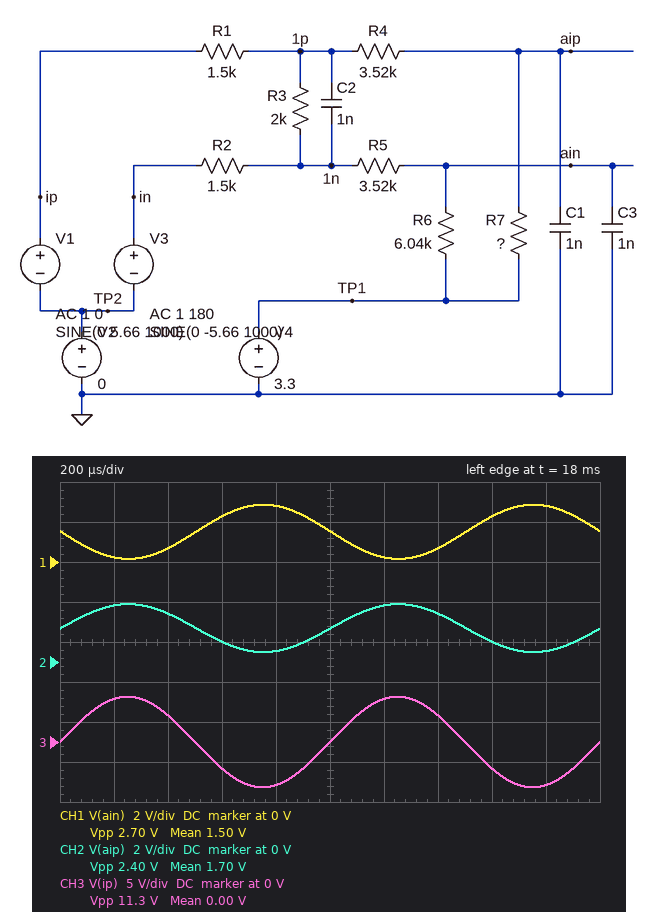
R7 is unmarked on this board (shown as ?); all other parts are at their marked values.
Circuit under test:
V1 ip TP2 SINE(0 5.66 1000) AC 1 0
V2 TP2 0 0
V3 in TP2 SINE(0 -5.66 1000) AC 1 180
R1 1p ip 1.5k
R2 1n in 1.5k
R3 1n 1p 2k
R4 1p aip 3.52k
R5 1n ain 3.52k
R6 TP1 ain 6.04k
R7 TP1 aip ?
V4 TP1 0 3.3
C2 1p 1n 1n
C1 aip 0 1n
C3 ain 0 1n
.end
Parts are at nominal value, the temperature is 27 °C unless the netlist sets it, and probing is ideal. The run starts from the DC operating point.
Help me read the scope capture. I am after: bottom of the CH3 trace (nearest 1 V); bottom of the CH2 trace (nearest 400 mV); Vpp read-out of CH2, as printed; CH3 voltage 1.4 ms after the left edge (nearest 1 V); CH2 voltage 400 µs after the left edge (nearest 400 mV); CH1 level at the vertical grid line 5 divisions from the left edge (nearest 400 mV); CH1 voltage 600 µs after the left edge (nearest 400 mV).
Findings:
-6 V
400 mV
2.40 V
3 V
2.4 V
1.6 V
2.4 V
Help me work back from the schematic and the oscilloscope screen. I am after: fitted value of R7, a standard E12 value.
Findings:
4.7 kΩ
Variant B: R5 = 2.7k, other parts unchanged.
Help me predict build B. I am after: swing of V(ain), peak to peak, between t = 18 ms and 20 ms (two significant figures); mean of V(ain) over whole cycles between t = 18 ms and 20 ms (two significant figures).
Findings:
2.9 V
1.4 V
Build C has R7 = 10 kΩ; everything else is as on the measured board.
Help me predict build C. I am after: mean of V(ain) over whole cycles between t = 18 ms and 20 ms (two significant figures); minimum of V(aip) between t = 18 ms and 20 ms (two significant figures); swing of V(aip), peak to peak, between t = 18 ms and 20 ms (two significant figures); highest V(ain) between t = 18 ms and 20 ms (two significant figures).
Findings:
1.5 V
-490 mV
3.2 V
2.8 V
